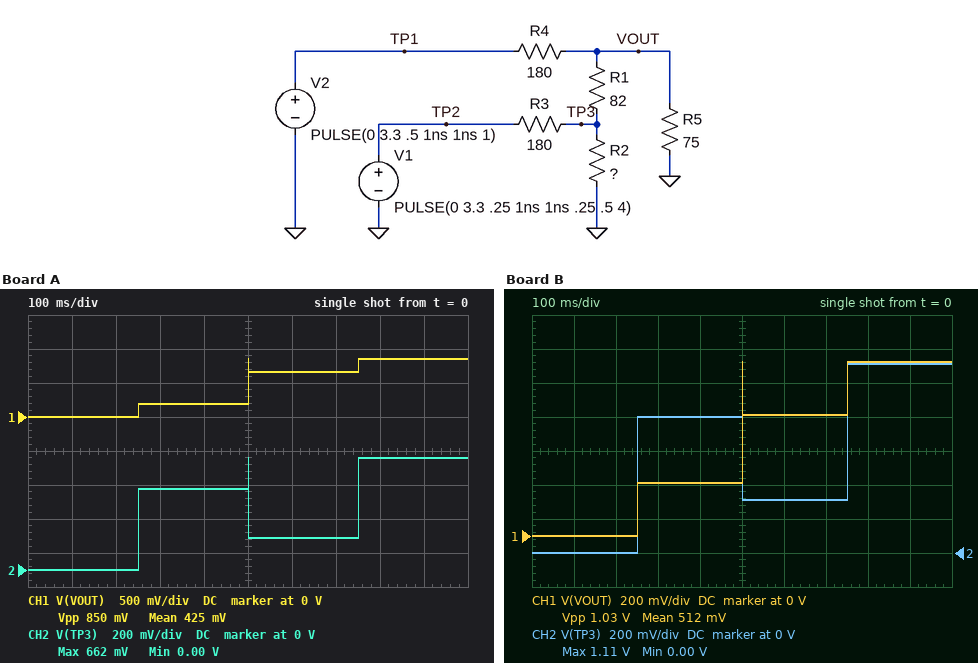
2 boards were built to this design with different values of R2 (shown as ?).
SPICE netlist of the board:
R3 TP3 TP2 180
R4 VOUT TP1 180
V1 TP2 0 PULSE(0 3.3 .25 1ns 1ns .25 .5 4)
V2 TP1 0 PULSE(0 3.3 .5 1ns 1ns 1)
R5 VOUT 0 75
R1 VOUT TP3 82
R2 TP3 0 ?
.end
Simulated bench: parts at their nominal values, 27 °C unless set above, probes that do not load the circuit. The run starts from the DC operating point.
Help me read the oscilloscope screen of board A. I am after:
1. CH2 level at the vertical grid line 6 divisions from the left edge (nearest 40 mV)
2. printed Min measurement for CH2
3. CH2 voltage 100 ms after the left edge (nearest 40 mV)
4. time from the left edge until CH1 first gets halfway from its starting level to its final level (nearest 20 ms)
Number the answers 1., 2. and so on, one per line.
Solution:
1. 200 mV
2. 0.00 V
3. 0 V
4. 500 ms
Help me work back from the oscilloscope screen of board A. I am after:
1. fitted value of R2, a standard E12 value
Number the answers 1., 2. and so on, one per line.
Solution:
1. 39 Ω
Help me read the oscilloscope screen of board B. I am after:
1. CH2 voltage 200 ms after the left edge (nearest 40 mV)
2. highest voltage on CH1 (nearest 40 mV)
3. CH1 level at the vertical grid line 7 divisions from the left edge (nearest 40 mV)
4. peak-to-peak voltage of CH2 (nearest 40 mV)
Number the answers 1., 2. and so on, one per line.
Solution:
1. 0 V
2. 1.04 V
3. 720 mV
4. 1.12 V
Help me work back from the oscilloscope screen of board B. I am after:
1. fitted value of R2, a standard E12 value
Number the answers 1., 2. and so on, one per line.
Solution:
1. 100 Ω
